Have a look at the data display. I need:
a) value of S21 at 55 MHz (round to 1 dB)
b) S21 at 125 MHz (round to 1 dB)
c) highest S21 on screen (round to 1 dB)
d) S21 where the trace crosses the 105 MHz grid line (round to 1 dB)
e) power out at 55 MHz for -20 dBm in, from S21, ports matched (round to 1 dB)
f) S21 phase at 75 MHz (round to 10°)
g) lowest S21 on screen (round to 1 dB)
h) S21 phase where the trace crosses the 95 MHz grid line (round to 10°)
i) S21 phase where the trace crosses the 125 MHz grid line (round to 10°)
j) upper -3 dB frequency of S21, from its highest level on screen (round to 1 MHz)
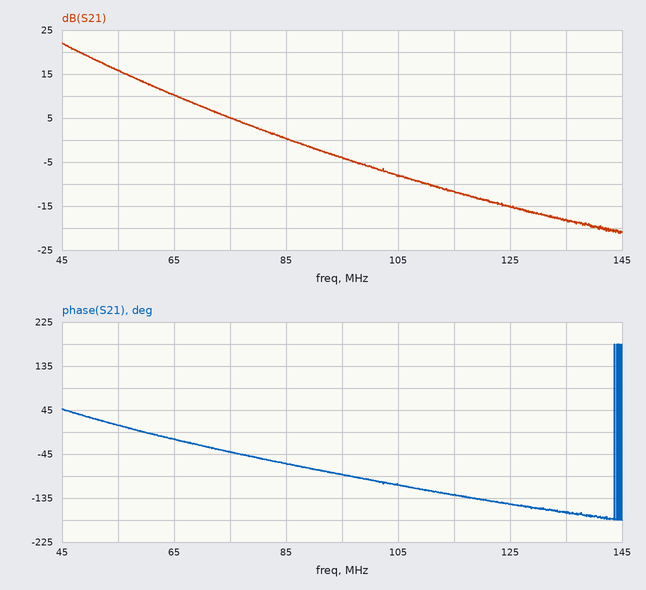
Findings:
16 dB
-15 dB
22 dB
-8 dB
-4 dBm
-40°
-21 dB
-90°
-150°
50 MHz
